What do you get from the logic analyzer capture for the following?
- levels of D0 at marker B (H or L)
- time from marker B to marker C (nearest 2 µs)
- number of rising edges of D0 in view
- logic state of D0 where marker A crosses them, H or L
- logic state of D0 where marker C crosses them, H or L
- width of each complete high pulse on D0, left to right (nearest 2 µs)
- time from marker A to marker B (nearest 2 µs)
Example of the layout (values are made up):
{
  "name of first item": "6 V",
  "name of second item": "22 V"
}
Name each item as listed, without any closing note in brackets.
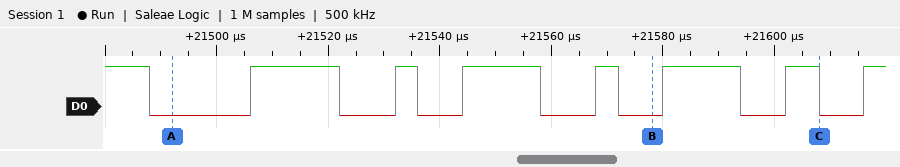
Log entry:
{
  "levels of D0 at marker B": "D0=L",
  "time from marker B to marker C": "30 µs",
  "number of rising edges of D0 in view": "7",
  "logic state of D0 where marker A crosses them, H or L": "D0=L",
  "logic state of D0 where marker C crosses them, H or L": "D0=L",
  "width of each complete high pulse on D0, left to right": "16 µs, 4 µs, 14 µs, 4 µs, 14 µs, 6 µs",
  "time from marker A to marker B": "86 µs"
}
